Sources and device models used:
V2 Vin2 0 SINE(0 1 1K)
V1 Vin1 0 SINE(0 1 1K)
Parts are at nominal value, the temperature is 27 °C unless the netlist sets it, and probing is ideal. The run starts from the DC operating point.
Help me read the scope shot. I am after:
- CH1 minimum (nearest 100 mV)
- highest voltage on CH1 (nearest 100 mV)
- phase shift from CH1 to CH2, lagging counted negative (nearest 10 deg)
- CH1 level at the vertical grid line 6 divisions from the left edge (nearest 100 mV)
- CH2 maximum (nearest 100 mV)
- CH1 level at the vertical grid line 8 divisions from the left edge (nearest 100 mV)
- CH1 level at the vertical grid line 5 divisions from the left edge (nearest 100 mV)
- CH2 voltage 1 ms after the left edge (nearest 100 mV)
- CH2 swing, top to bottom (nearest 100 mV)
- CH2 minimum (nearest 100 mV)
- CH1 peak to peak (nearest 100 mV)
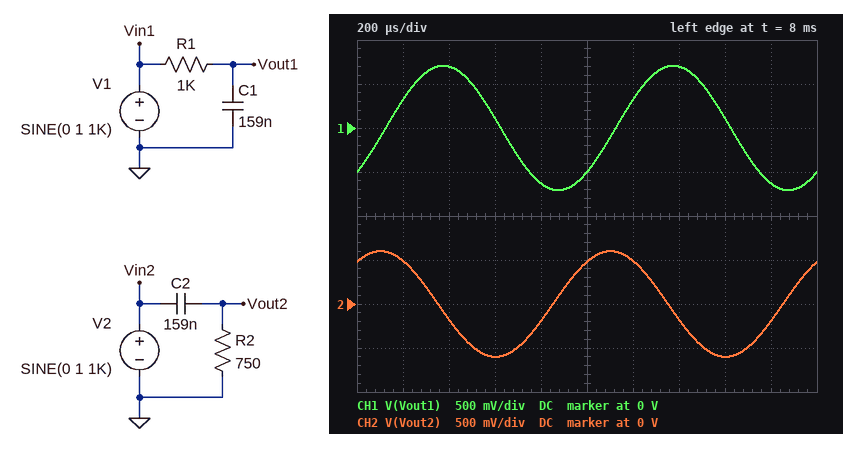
-700 mV
700 mV
100 deg
300 mV
600 mV
100 mV
-500 mV
500 mV
1.2 V
-600 mV
1.4 V
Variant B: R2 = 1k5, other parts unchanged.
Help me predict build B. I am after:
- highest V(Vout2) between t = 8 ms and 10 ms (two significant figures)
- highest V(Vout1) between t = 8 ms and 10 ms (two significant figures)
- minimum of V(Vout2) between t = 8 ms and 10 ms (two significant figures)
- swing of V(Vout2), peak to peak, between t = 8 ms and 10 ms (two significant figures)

830 mV
710 mV
-830 mV
1.7 V
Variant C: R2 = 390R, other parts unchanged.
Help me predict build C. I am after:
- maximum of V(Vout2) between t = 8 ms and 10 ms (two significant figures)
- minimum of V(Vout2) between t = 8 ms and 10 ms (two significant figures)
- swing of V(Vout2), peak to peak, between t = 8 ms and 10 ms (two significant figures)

360 mV
-360 mV
730 mV
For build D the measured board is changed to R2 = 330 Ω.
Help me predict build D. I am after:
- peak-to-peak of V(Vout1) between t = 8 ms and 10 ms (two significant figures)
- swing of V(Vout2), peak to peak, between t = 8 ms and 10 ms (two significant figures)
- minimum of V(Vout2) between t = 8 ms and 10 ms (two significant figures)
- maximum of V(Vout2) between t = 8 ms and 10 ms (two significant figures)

1.4 V
630 mV
-310 mV
310 mV
